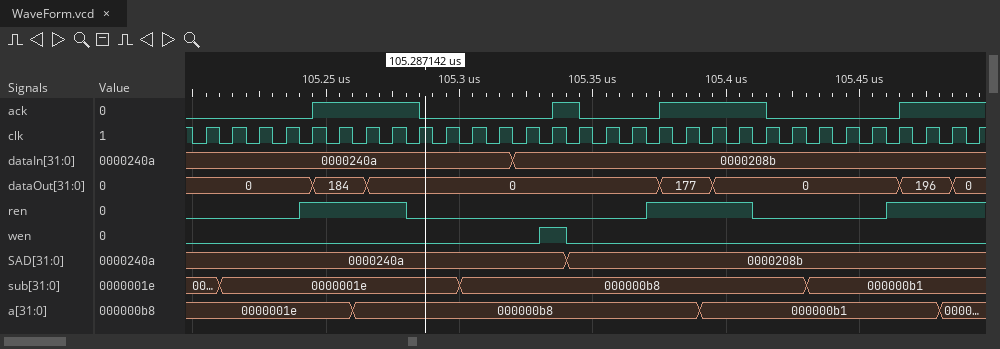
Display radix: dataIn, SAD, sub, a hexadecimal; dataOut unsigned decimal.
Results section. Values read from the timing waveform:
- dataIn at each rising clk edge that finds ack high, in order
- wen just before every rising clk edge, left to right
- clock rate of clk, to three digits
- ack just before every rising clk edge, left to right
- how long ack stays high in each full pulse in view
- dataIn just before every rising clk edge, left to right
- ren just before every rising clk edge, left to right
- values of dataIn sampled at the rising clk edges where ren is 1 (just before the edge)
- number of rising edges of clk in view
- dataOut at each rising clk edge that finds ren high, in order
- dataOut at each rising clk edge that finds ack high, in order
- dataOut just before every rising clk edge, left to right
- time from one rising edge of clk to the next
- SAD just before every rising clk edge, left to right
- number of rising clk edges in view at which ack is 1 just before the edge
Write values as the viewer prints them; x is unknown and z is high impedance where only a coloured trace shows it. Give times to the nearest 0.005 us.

0000240a, 0000240a, 0000240a, 0000240a, 0000208b, 0000208b, 0000208b, 0000208b, 0000208b, 0000208b, 0000208b, 0000208b
0 0 0 0 0 0 0 0 0 0 0 0 0 1 0 0 0 0 0 0 0 0 0 0 0 0 0 0 0 0
100 MHz
0 0 0 0 0 1 1 1 1 0 0 0 0 0 1 0 0 0 1 1 1 1 0 0 0 0 0 1 1 1
0.04 us, 0.01 us, 0.04 us
0000240a, 0000240a, 0000240a, 0000240a, 0000240a, 0000240a, 0000240a, 0000240a, 0000240a, 0000240a, 0000240a, 0000240a, 0000208b, 0000208b, 0000208b, 0000208b, 0000208b, 0000208b, 0000208b, 0000208b, 0000208b, 0000208b, 0000208b, 0000208b, 0000208b, 0000208b, 0000208b, 0000208b, 0000208b, 0000208b
0 0 0 0 1 1 1 1 0 0 0 0 0 0 0 0 0 1 1 1 1 0 0 0 0 0 1 1 1 1
0000240a, 0000240a, 0000240a, 0000240a, 0000208b, 0000208b, 0000208b, 0000208b, 0000208b, 0000208b, 0000208b, 0000208b
30
0, 184, 184, 0, 0, 177, 177, 0, 0, 196, 196, 0
184, 184, 0, 0, 0, 177, 177, 0, 0, 196, 196, 0
0, 0, 0, 0, 0, 184, 184, 0, 0, 0, 0, 0, 0, 0, 0, 0, 0, 0, 177, 177, 0, 0, 0, 0, 0, 0, 0, 196, 196, 0
0.01 us
0000240a, 0000240a, 0000240a, 0000240a, 0000240a, 0000240a, 0000240a, 0000240a, 0000240a, 0000240a, 0000240a, 0000240a, 0000240a, 0000240a, 0000208b, 0000208b, 0000208b, 0000208b, 0000208b, 0000208b, 0000208b, 0000208b, 0000208b, 0000208b, 0000208b, 0000208b, 0000208b, 0000208b, 0000208b, 0000208b
12
